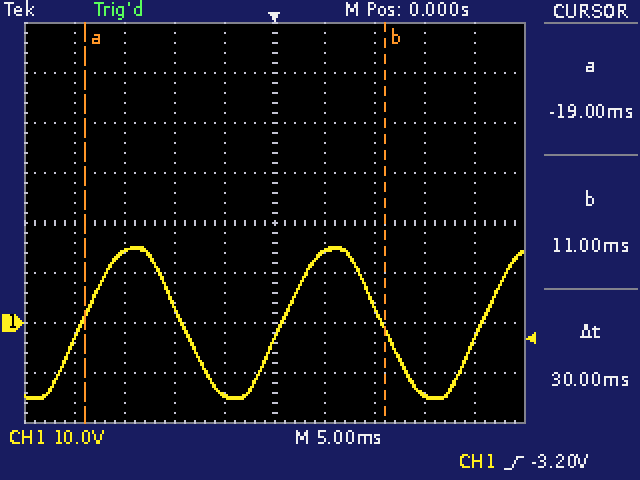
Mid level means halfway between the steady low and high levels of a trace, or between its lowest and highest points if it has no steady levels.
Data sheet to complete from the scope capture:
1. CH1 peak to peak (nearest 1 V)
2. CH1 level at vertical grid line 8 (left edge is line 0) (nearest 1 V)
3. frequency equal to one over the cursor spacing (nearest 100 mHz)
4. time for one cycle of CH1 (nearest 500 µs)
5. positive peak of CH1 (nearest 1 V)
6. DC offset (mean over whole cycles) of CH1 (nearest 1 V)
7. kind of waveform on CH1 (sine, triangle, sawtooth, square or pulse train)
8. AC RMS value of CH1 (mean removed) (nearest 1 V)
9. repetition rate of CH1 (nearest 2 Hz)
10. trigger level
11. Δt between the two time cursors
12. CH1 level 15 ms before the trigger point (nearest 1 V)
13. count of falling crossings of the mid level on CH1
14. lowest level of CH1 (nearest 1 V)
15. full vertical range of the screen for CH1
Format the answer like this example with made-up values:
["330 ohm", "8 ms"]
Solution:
["30 V", "-14 V", "33.3 Hz", "20.0 ms", "15 V", "0 V", "sine", "11 V", "50 Hz", "-3.20 V", "30 ms", "14 V", "2", "-15 V", "80 V"]
